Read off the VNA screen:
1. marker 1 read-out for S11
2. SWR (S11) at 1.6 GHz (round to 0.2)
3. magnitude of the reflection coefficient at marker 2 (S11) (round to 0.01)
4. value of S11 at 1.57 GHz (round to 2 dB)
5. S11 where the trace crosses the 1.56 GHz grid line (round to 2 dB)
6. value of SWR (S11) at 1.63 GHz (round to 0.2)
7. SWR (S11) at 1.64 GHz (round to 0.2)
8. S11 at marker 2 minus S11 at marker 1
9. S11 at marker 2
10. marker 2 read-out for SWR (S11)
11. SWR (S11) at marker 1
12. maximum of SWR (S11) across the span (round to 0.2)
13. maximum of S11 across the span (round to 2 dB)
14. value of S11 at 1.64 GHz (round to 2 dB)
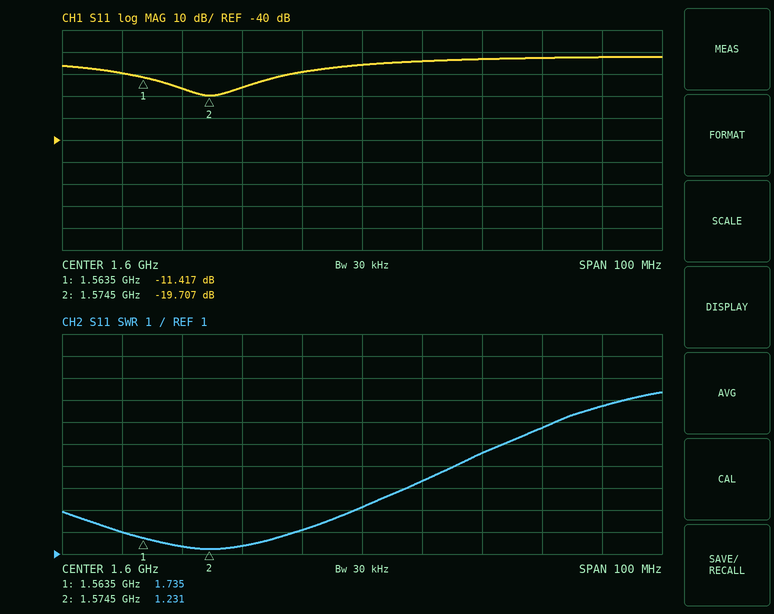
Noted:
-11.417 dB
3.2
0.10
-16 dB
-10 dB
6.8
7.8
-8.290 dB
-19.707 dB
1.231
1.735
8.4
-2 dB
-2 dB
